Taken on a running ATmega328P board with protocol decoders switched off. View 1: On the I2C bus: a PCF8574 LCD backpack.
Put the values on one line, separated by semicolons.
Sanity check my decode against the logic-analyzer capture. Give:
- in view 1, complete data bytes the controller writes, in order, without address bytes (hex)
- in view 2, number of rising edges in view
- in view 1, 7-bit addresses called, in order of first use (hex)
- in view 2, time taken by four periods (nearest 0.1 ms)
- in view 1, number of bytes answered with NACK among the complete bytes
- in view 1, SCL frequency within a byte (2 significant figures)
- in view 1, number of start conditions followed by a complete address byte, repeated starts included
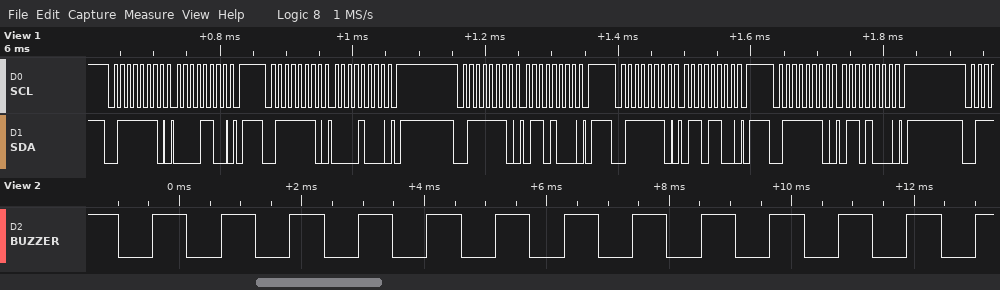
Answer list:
0C 08 68 6C 68; 13; 0x3F; 4.5 ms; 0; 100 kHz; 5
